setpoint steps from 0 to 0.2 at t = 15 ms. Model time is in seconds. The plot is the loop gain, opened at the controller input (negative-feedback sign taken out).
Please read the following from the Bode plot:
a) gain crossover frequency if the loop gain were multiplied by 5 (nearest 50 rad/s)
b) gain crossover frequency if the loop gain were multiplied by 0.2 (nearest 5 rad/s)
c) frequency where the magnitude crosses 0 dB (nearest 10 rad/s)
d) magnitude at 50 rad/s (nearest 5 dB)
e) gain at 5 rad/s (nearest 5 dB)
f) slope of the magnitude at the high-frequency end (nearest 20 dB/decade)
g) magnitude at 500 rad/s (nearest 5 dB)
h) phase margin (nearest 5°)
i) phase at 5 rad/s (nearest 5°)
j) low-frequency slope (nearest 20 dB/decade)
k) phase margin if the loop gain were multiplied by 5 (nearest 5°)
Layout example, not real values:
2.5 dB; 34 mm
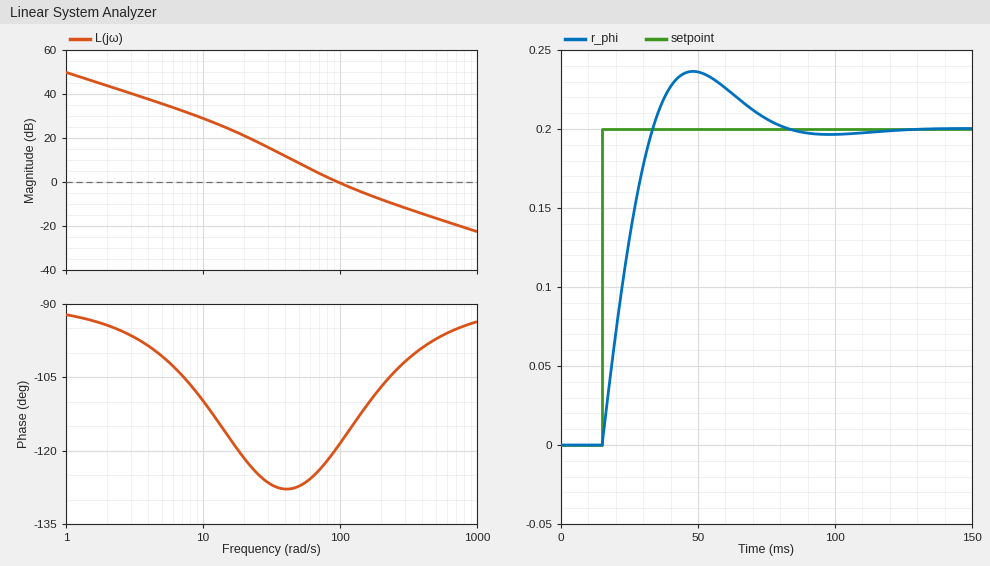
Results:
400 rad/s; 35 rad/s; 100 rad/s; 10 dB; 35 dB; -20 dB/decade; -15 dB; 60°; -100°; -20 dB/decade; 80°
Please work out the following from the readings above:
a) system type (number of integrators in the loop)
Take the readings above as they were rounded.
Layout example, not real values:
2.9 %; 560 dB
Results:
1
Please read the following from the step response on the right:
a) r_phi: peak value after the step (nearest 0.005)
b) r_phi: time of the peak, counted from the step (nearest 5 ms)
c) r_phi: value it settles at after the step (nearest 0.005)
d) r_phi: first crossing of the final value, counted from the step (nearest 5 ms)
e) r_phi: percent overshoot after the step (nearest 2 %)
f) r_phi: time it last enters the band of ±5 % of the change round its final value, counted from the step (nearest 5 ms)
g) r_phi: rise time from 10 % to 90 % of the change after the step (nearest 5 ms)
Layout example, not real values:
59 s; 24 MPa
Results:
0.235; 35 ms; 0.200; 20 ms; 18 %; 55 ms; 15 ms
